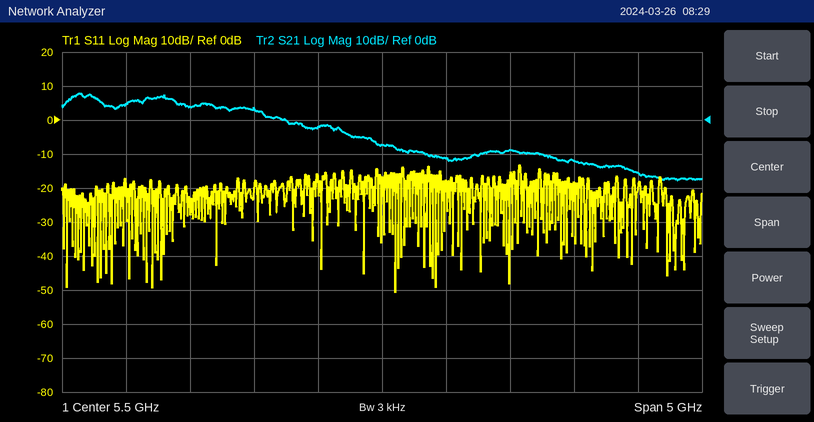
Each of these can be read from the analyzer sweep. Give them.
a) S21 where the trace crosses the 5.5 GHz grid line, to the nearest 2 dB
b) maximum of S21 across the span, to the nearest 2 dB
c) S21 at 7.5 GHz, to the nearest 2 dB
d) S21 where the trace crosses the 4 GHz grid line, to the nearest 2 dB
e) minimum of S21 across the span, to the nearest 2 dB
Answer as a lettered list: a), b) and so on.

a) -8 dB
b) 8 dB
c) -16 dB
d) 4 dB
e) -18 dB
